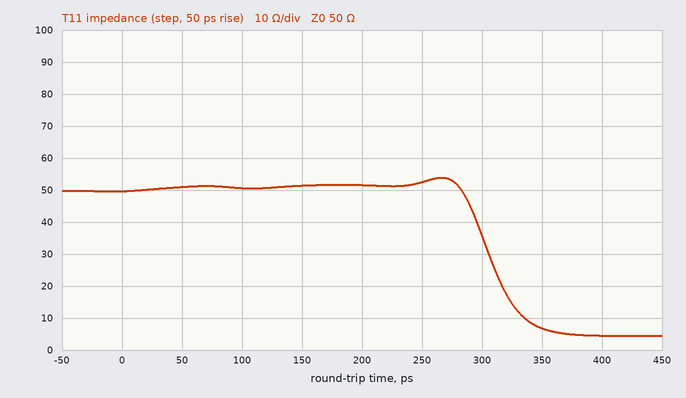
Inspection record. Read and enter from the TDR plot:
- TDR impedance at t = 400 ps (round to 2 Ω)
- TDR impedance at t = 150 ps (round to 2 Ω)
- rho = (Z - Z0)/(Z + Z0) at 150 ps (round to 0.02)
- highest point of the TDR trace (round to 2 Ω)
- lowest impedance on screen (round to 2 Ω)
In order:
4 Ω
52 Ω
+0.02
54 Ω
4 Ω
